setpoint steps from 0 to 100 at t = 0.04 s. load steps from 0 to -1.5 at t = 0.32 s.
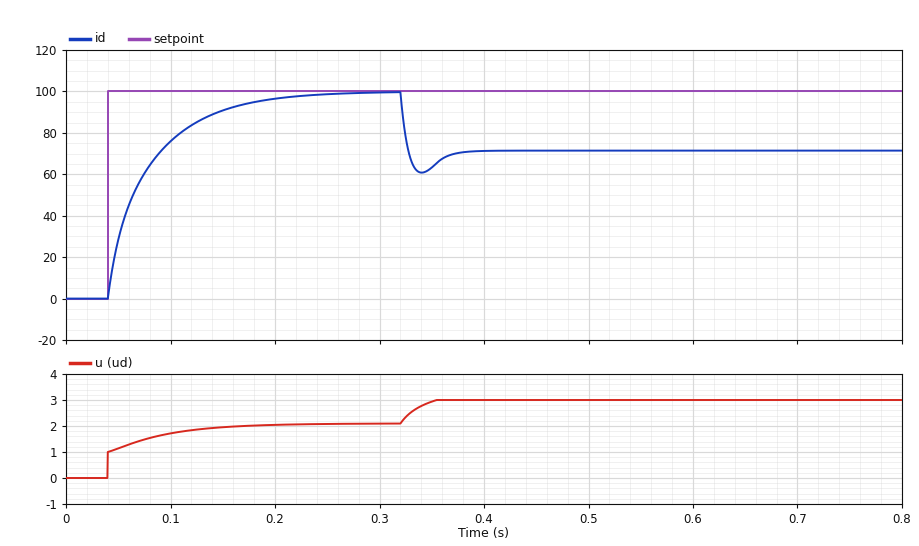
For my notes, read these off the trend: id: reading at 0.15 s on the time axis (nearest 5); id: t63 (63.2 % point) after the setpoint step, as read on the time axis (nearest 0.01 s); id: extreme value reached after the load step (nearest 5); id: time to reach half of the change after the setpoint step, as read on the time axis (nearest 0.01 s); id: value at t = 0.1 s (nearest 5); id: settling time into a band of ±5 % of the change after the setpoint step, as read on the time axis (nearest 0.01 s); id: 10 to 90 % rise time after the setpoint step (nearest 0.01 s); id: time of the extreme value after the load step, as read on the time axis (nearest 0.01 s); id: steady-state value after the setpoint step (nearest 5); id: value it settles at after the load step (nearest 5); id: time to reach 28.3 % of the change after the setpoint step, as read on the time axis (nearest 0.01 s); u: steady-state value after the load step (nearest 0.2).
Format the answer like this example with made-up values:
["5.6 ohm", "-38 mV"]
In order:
["90", "0.08 s", "60", "0.06 s", "75", "0.18 s", "0.10 s", "0.34 s", "100", "70", "0.05 s", "3.0"]
